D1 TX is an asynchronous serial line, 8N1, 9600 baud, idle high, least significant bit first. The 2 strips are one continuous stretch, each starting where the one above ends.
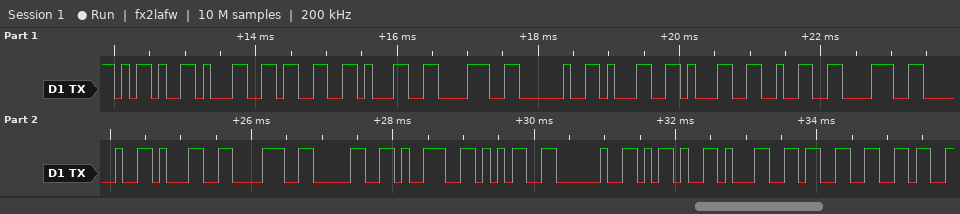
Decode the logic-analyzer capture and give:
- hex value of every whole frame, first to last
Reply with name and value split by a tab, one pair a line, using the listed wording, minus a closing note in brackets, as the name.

hex value of every whole frame, first to last	2D 31 33 31 38 20 31 31 32 38 20 31 38 30 39 35 20 2D 31 33 36
